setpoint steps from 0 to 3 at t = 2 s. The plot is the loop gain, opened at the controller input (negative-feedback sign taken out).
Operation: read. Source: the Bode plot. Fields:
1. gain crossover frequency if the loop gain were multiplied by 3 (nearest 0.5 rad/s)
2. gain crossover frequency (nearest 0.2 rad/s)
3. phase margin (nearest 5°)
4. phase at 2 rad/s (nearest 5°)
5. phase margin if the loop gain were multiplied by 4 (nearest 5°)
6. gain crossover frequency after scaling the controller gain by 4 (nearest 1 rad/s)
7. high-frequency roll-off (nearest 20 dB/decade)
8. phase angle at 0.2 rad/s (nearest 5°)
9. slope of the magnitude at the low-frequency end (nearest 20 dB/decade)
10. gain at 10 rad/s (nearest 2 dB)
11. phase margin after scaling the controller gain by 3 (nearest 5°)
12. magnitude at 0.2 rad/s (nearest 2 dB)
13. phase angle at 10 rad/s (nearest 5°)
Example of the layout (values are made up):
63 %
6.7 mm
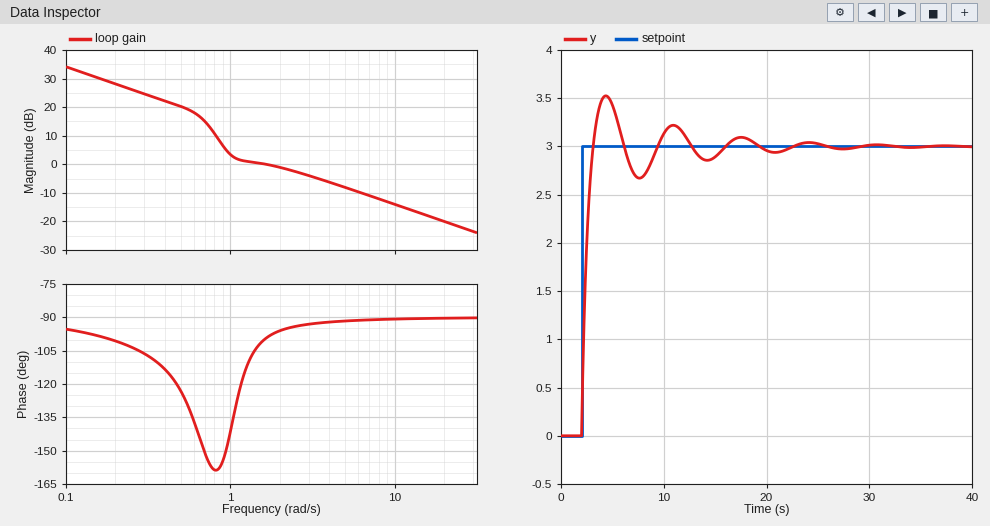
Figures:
6.0 rad/s
1.6 rad/s
80°
-95°
90°
8 rad/s
-20 dB/decade
-100°
-20 dB/decade
-14 dB
90°
28 dB
-90°
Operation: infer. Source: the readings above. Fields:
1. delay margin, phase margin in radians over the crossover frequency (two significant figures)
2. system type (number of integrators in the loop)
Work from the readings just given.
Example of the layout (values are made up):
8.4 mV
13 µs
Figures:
0.87 s
1
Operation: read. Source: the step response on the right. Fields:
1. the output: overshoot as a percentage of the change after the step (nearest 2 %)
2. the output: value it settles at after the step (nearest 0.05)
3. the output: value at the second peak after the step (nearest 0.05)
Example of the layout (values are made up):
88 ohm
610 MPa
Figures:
18 %
3.00
3.20
